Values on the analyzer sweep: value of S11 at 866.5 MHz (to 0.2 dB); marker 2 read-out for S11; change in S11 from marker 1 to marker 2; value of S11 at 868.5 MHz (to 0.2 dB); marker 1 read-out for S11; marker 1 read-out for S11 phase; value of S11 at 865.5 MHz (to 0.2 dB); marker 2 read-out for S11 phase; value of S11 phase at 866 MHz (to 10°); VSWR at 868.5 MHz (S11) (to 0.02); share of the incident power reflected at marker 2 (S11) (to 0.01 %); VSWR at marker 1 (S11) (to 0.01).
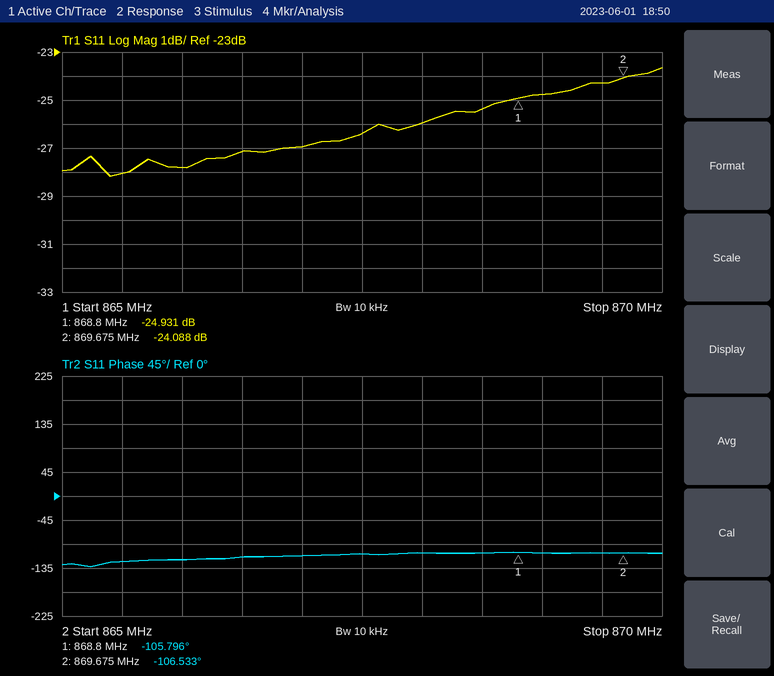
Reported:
-27.2 dB
-24.088 dB
0.843 dB
-25.4 dB
-24.931 dB
-105.796°
-28.0 dB
-106.533°
-120°
1.12
0.39 %
1.12
